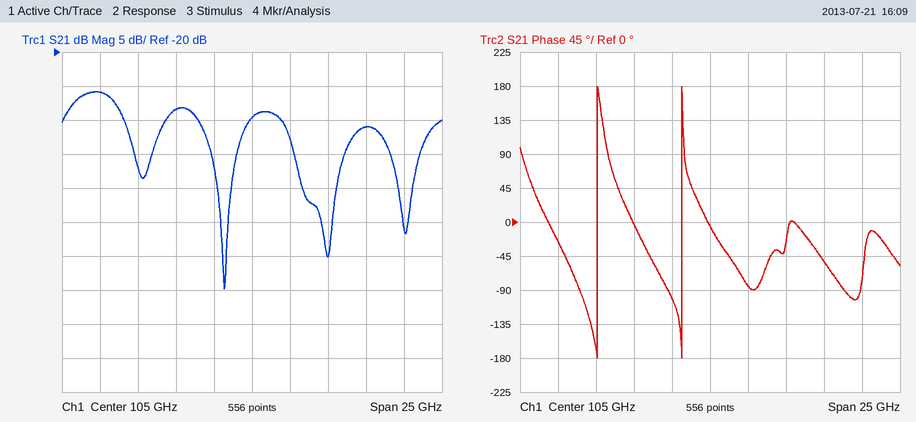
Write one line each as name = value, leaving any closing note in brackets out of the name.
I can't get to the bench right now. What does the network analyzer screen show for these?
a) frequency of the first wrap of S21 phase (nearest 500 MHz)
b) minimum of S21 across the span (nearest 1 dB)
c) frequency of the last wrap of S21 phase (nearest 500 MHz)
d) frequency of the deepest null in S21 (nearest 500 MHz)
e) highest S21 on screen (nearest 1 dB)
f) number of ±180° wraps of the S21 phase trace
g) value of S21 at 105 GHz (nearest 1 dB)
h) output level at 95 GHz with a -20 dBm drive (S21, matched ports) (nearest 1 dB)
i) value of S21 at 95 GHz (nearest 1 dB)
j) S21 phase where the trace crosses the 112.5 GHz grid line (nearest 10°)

frequency of the first wrap of S21 phase = 97.5 GHz
minimum of S21 across the span = -55 dB
frequency of the last wrap of S21 phase = 103.0 GHz
frequency of the deepest null in S21 = 103.0 GHz
highest S21 on screen = -26 dB
number of ±180° wraps of the S21 phase trace = 2
value of S21 at 105 GHz = -30 dB
output level at 95 GHz with a -20 dBm drive (S21, matched ports) = -46 dBm
value of S21 at 95 GHz = -26 dB
S21 phase where the trace crosses the 112.5 GHz grid line = -50°
